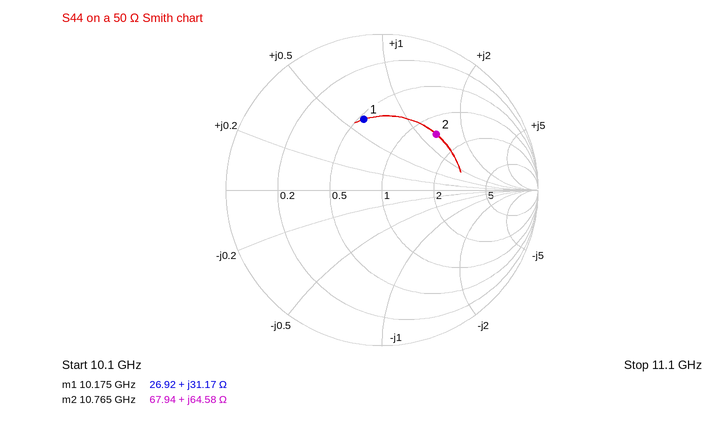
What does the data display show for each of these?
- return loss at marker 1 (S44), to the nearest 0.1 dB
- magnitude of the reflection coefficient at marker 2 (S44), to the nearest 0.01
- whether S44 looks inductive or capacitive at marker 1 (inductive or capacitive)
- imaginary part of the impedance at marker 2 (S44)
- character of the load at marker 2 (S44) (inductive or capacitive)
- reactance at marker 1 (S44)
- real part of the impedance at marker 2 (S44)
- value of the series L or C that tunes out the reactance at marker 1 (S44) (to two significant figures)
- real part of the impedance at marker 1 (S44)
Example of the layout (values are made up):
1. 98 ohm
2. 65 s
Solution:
1. 6.6 dB
2. 0.50
3. inductive
4. +64.58 Ω
5. inductive
6. +31.17 Ω
7. 67.94 Ω
8. 500 fF
9. 26.92 Ω
